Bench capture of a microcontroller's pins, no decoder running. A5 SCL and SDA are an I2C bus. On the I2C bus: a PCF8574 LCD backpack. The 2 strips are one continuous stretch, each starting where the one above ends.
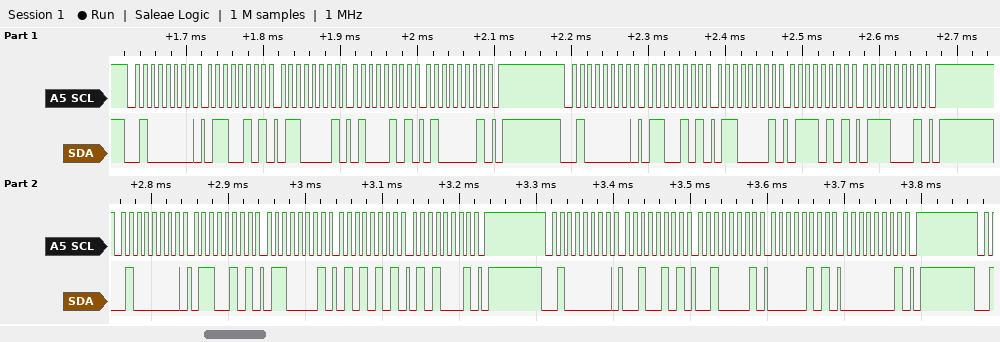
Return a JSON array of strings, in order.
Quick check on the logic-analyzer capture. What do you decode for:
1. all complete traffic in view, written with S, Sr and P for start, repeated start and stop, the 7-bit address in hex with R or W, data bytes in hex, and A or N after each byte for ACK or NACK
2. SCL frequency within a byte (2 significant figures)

["S 20W A 65 A 61 A 45 A 41 A P S 20W A 65 A 61 A 75 A 71 A P S 20W A 65 A 61 A 55 A 51 A P S 20W A 25 A 21 A 05 A 01 A P", "100 kHz"]
